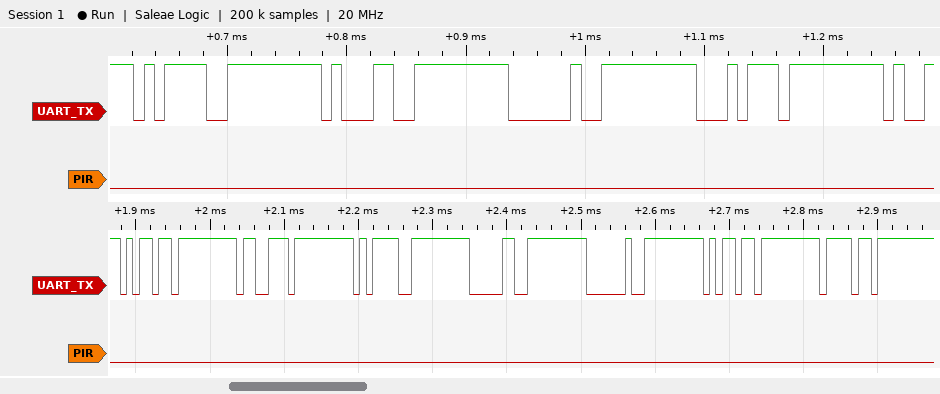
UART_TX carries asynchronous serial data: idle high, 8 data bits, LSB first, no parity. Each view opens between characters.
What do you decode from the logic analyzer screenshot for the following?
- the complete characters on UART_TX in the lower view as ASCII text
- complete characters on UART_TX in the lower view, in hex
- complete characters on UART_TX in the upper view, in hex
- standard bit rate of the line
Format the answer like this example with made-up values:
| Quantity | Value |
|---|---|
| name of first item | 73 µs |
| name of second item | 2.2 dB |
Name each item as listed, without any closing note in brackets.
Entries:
| Quantity | Value |
|---|---|
| the complete characters on UART_TX in the lower view as ASCII text | "ms=0 mo" |
| complete characters on UART_TX in the lower view, in hex | 6D, 73, 3D, 30, 20, 6D, 6F |
| complete characters on UART_TX in the upper view, in hex | 3D, 31, 20, 74 |
| standard bit rate of the line | 115200 baud |
